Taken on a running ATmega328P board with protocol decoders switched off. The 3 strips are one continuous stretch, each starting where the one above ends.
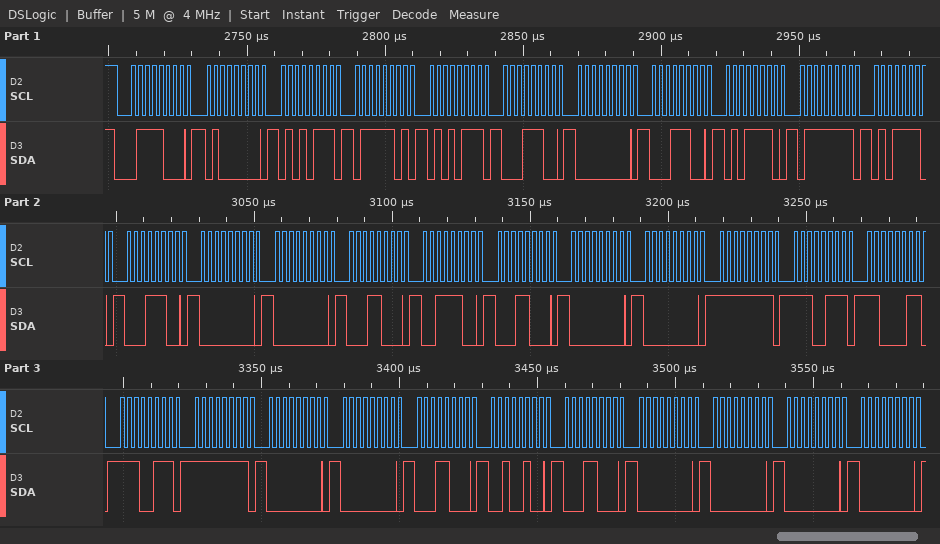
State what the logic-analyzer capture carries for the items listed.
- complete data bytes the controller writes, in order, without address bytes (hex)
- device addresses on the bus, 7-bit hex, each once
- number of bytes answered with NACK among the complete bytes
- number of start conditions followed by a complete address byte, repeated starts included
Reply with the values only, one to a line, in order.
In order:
40 57 7D 57 1C 00 1C 5E 7F 5E 1C 00 00 18 3C 18 00 00 FF E7 C3 E7 FF 00 00 18 24 18 00 00 00 00
0x3C
0
1
